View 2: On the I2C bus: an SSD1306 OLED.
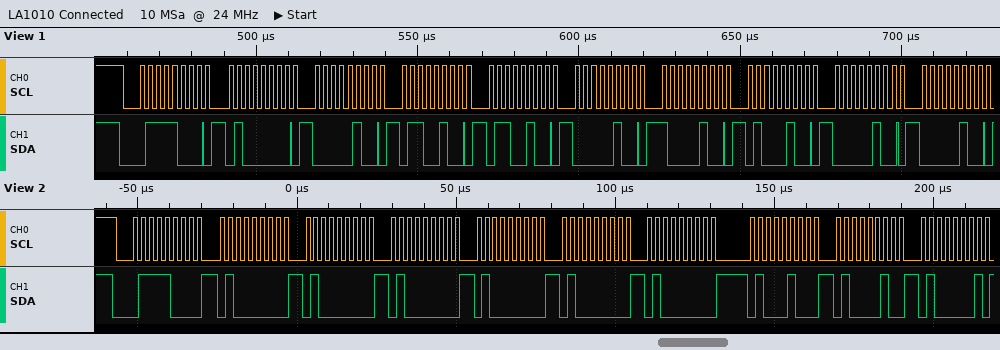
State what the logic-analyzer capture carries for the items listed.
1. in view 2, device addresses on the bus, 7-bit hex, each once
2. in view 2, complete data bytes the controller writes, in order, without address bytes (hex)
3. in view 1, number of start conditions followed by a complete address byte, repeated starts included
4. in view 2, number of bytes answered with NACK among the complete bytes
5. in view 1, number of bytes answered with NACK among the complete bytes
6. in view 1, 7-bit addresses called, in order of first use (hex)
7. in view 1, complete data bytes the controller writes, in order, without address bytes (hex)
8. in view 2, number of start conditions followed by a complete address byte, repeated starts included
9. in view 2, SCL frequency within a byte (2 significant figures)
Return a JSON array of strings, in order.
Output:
["0x3C", "40 40 40 40 40 40 44 42 41", "1", "0", "0", "0x3C", "40 04 64 64 04 84 44 04 04", "1", "400 kHz"]
